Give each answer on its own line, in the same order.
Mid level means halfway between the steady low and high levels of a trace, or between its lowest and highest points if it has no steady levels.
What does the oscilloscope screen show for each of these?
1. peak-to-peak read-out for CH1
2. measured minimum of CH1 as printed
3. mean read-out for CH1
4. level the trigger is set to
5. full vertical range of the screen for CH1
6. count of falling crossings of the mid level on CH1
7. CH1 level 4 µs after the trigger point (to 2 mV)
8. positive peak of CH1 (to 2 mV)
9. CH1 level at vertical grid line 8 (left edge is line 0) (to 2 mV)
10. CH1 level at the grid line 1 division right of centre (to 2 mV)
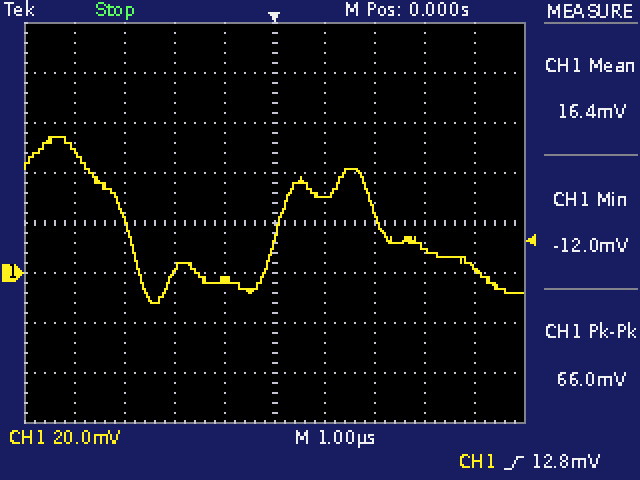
66.0 mV
-12.0 mV
16.4 mV
12.8 mV
160 mV
2
2 mV
54 mV
10 mV
30 mV
